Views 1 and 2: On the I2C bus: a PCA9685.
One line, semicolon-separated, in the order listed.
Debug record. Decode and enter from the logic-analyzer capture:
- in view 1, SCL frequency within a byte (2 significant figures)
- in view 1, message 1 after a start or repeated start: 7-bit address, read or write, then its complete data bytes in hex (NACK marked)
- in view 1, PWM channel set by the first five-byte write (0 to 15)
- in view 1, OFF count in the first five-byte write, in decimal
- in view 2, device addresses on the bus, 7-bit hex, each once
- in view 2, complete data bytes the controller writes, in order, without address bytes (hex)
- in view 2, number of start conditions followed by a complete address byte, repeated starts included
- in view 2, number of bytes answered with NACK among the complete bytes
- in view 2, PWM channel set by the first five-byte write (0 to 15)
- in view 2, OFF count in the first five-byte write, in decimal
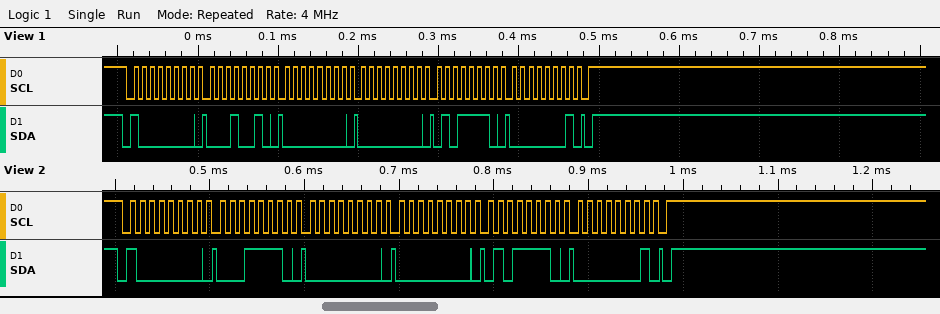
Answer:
100 kHz; 0x40 write: 12 00 00 5E 01; 3; 350; 0x40; 1E 00 00 5E 01; 1; 0; 6; 350
